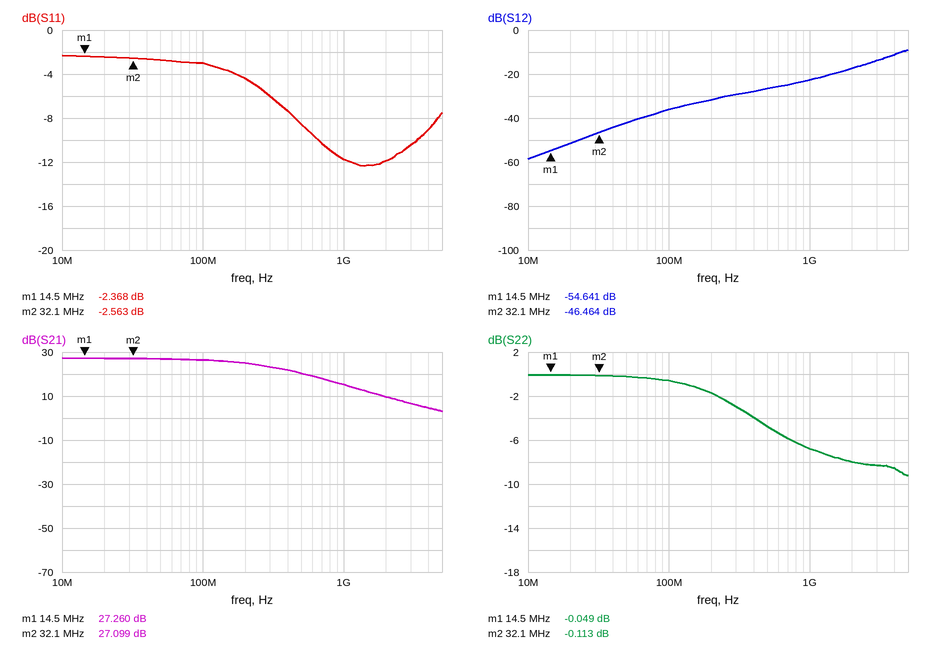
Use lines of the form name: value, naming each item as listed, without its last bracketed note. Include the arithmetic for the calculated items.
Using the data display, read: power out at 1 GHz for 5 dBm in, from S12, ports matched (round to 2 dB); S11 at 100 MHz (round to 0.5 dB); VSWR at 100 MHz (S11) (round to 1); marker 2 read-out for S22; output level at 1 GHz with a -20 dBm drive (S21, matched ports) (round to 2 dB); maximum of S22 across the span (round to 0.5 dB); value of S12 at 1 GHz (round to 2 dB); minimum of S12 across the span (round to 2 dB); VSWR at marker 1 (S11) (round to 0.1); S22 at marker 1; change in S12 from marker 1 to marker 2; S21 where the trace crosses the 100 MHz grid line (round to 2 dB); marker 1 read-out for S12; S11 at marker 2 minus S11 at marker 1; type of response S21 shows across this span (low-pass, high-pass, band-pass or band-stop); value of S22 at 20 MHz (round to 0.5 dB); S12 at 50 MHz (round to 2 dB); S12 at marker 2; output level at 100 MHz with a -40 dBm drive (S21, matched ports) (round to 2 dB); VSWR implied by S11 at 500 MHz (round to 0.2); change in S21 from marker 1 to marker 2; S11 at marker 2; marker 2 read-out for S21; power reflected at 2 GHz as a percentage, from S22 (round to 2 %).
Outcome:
power out at 1 GHz for 5 dBm in, from S12, ports matched: 5 dBm + (-22 dB) = -18 dBm
S11 at 100 MHz: -3.0 dB
VSWR at 100 MHz (S11): |Γ| = 10^(-3/20) = 0.7079; VSWR = (1 + 0.7079)/(1 − 0.7079) ≈ 6
marker 2 read-out for S22: -0.113 dB
output level at 1 GHz with a -20 dBm drive (S21, matched ports): -20 dBm + (16 dB) = -4 dBm
maximum of S22 across the span: 0.0 dB
value of S12 at 1 GHz: -22 dB
minimum of S12 across the span: -58 dB
VSWR at marker 1 (S11): (1 + 0.7614)/(1 − 0.7614) ≈ 7.4
S22 at marker 1: -0.049 dB
change in S12 from marker 1 to marker 2: -46.464 − (-54.641) = 8.177 dB
S21 where the trace crosses the 100 MHz grid line: 26 dB
marker 1 read-out for S12: -54.641 dB
S11 at marker 2 minus S11 at marker 1: -2.563 − (-2.368) = -0.195 dB
type of response S21 shows across this span: low-pass
value of S22 at 20 MHz: 0.0 dB
S12 at 50 MHz: -42 dB
S12 at marker 2: -46.464 dB
output level at 100 MHz with a -40 dBm drive (S21, matched ports): -40 dBm + (26 dB) = -14 dBm
VSWR implied by S11 at 500 MHz: |Γ| = 10^(-8.5/20) = 0.3758; VSWR = (1 + 0.3758)/(1 − 0.3758) ≈ 2.2
change in S21 from marker 1 to marker 2: 27.099 − (27.26) = -0.161 dB
S11 at marker 2: -2.563 dB
marker 2 read-out for S21: 27.099 dB
power reflected at 2 GHz as a percentage, from S22: 10^(-8/10) ≈ 16 %
